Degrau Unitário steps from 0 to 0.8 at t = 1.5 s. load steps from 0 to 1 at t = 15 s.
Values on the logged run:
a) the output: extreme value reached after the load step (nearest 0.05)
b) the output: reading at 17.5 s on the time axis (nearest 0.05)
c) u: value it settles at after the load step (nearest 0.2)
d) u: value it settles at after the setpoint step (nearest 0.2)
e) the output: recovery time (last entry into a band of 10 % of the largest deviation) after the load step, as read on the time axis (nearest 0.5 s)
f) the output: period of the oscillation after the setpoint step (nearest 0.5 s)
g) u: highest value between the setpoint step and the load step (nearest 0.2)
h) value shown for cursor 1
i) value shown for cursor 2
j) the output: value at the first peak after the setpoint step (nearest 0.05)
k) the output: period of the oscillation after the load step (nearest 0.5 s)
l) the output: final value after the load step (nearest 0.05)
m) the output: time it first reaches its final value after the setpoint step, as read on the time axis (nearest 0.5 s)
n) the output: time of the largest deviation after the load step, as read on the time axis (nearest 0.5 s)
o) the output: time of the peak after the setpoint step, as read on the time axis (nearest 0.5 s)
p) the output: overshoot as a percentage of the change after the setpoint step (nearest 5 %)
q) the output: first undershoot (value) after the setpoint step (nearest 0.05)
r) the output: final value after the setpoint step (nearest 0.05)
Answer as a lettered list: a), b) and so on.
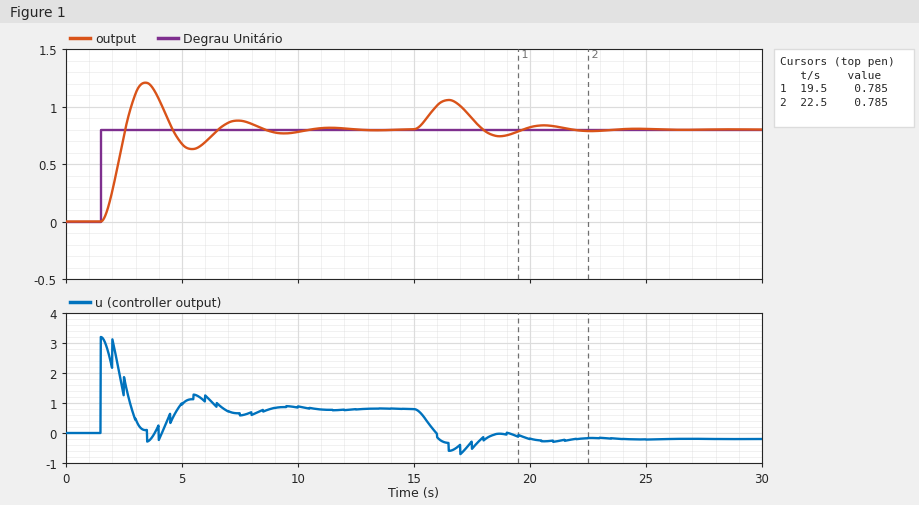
a) 1.05
b) 0.90
c) -0.2
d) 0.8
e) 21.0 s
f) 4.0 s
g) 3.2
h) 0.785
i) 0.785
j) 1.20
k) 4.0 s
l) 0.80
m) 2.5 s
n) 16.5 s
o) 3.5 s
p) 50 %
q) 0.65
r) 0.80
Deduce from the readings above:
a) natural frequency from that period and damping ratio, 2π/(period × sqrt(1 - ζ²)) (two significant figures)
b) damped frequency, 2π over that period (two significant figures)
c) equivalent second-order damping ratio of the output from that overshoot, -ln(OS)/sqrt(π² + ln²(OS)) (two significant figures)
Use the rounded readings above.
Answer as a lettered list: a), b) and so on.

a) 1.6 rad/s
b) 1.6 rad/s
c) 0.22
